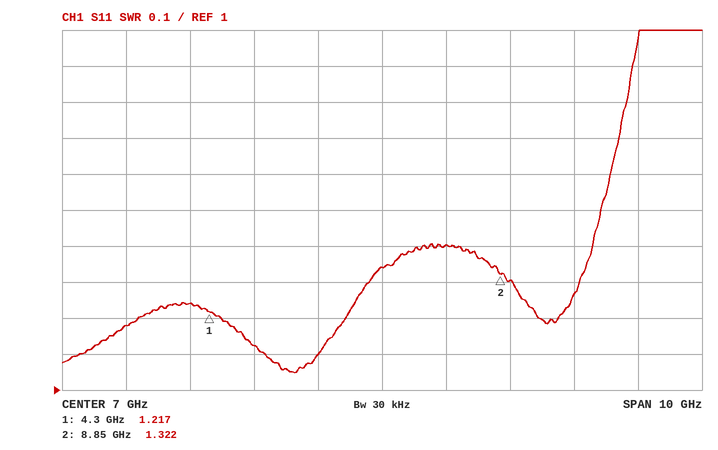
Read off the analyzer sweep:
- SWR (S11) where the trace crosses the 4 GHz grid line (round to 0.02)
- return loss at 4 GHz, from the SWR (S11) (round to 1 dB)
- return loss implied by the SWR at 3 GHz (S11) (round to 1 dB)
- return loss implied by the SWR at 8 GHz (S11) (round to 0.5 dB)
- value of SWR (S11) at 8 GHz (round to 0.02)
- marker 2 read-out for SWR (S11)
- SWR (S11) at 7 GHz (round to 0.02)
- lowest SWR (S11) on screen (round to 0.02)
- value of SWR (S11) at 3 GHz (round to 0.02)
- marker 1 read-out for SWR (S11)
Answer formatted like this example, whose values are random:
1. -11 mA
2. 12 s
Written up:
1. 1.24
2. 19 dB
3. 22 dB
4. 15.5 dB
5. 1.40
6. 1.322
7. 1.34
8. 1.04
9. 1.18
10. 1.217
